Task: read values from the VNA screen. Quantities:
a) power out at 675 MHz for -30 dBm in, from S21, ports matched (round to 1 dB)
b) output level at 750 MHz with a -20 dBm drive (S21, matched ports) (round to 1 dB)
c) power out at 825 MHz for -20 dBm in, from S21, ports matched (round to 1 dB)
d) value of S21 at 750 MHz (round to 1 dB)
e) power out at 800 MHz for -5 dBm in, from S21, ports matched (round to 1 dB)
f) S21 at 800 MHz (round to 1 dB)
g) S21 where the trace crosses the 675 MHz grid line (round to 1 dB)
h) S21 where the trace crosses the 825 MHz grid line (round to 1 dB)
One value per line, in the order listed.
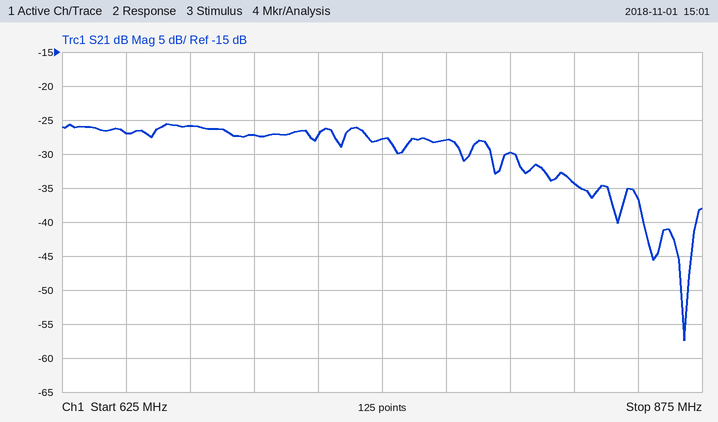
-56 dBm
-48 dBm
-54 dBm
-28 dB
-35 dBm
-30 dB
-26 dB
-34 dB
